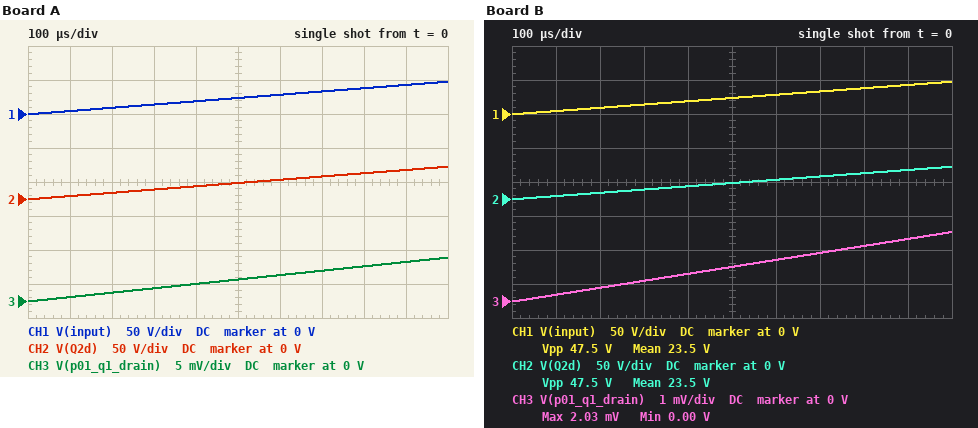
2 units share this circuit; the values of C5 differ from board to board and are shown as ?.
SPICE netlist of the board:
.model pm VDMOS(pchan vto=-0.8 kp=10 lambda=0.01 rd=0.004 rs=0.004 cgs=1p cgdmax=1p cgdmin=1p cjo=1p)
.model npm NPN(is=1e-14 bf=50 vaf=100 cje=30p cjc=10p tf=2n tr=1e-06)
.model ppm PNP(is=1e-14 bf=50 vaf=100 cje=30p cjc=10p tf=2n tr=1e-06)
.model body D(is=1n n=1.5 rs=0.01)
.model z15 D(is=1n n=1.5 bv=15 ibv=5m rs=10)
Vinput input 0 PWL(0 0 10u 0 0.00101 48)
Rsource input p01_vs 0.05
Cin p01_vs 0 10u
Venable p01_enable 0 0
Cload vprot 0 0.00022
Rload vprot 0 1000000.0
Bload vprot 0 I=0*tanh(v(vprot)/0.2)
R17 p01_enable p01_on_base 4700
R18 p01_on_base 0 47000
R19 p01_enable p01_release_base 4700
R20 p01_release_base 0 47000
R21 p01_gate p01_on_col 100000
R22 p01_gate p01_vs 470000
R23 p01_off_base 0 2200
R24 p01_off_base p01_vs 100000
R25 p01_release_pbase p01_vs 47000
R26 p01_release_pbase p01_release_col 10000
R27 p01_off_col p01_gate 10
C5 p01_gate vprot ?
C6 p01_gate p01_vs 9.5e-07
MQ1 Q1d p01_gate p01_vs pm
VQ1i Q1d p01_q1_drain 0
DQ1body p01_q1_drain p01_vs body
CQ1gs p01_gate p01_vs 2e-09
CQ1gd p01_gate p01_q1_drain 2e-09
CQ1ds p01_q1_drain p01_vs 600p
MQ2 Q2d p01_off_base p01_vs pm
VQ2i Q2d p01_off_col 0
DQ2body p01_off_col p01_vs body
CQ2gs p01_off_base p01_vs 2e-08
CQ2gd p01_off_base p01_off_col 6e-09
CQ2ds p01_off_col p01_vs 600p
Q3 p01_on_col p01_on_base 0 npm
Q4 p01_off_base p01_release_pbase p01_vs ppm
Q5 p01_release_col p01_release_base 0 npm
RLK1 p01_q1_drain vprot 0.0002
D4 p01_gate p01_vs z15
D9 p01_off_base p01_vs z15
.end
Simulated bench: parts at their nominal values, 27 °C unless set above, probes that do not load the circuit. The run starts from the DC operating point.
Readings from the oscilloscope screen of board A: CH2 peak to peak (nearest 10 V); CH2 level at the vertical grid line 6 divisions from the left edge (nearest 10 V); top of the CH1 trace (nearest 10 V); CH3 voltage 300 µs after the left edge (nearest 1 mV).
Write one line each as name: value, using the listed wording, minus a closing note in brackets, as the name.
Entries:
CH2 peak to peak: 50 V
CH2 level at the vertical grid line 6 divisions from the left edge: 30 V
top of the CH1 trace: 50 V
CH3 voltage 300 µs after the left edge: 2 mV
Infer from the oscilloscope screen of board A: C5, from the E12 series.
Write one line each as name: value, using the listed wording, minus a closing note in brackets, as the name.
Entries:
C5, from the E12 series: 27 nF
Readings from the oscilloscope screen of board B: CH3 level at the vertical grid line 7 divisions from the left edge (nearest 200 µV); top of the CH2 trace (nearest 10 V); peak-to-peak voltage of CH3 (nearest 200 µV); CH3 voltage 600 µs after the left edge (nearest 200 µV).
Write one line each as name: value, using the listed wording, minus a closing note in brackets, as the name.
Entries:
CH3 level at the vertical grid line 7 divisions from the left edge: 1.4 mV
top of the CH2 trace: 50 V
peak-to-peak voltage of CH3: 2.0 mV
CH3 voltage 600 µs after the left edge: 1.2 mV
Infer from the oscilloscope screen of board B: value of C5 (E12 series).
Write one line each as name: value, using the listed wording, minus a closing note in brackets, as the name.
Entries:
value of C5: 6.8 nF
